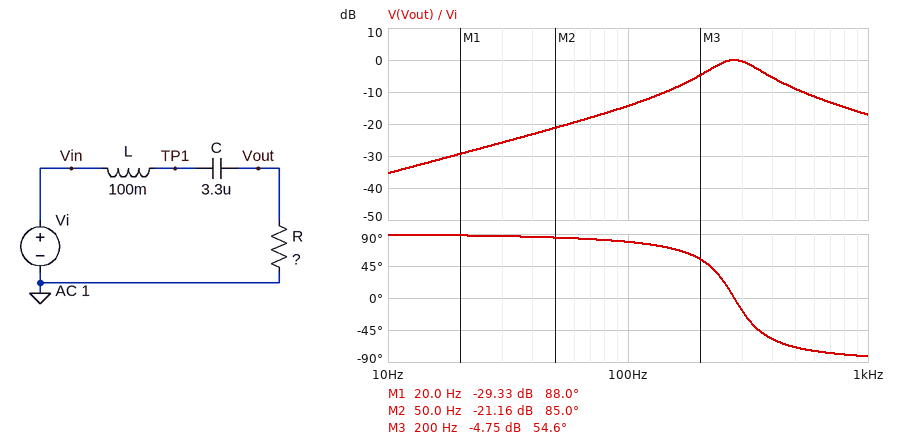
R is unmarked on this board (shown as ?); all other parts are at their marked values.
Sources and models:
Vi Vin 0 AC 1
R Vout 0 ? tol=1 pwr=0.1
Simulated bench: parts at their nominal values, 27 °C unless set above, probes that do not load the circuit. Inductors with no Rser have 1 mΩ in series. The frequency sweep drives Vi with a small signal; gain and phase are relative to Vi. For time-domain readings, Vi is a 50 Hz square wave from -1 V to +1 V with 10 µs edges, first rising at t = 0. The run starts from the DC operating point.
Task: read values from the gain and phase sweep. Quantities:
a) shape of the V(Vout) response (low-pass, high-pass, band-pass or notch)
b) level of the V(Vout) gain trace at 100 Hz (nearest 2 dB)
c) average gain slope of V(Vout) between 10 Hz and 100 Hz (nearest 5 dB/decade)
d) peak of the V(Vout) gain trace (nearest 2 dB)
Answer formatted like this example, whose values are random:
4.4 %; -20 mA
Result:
band-pass; -14 dB; 20 dB/decade; 0 dB
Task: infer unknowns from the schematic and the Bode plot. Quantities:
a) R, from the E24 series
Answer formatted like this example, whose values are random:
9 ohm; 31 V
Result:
82 Ω
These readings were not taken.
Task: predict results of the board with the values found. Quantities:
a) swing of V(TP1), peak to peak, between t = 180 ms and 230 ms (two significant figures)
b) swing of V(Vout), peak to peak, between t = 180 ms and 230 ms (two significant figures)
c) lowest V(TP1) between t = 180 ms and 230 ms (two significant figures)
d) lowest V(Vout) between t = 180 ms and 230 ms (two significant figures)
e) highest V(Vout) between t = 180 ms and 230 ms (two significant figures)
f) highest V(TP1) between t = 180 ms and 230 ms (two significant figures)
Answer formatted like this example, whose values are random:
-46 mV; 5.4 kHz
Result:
4.1 V; 1.4 V; -2.1 V; -690 mV; 690 mV; 2.1 V
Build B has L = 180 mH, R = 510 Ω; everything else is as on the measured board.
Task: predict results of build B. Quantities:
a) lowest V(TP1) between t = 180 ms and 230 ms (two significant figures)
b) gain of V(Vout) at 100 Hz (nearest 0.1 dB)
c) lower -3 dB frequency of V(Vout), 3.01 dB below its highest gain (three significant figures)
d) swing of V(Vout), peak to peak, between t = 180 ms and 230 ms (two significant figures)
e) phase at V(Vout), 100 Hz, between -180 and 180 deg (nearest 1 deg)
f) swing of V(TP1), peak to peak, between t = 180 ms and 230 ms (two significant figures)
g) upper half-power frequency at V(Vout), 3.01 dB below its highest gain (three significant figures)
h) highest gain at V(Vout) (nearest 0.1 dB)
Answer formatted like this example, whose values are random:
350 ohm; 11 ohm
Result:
-1.2 V; -1.8 dB; 80.3 Hz; 3.0 V; 36 deg; 2.5 V; 531 Hz; 0 dB
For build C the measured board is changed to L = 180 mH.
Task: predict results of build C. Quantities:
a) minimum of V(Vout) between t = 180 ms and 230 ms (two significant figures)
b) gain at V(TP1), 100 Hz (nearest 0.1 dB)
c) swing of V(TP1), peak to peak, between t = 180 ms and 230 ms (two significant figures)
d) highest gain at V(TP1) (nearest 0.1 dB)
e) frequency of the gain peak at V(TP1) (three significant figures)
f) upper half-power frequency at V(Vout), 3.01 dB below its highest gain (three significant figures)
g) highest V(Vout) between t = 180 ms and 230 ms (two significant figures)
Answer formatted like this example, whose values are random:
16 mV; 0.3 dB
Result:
-500 mV; 2.2 dB; 4.2 V; 9.7 dB; 201 Hz; 246 Hz; 500 mV
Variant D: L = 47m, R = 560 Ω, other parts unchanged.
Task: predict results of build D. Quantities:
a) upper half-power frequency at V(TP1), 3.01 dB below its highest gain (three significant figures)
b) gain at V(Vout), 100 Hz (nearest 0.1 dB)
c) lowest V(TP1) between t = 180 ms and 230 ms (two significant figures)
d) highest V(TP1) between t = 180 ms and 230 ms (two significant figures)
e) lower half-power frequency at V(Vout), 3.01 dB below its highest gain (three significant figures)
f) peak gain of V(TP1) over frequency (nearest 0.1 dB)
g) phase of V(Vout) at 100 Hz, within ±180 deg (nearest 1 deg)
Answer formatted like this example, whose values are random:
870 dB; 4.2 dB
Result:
1.86 kHz; -2.2 dB; -1.1 V; 1.1 V; 82.5 Hz; 0.3 dB; 39 deg
